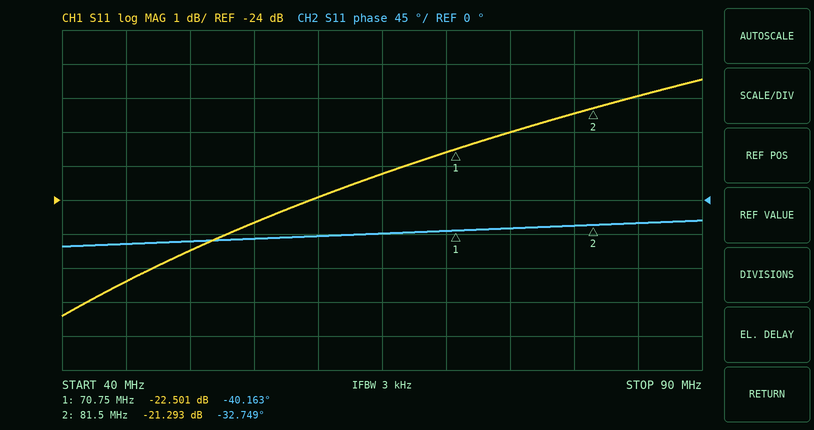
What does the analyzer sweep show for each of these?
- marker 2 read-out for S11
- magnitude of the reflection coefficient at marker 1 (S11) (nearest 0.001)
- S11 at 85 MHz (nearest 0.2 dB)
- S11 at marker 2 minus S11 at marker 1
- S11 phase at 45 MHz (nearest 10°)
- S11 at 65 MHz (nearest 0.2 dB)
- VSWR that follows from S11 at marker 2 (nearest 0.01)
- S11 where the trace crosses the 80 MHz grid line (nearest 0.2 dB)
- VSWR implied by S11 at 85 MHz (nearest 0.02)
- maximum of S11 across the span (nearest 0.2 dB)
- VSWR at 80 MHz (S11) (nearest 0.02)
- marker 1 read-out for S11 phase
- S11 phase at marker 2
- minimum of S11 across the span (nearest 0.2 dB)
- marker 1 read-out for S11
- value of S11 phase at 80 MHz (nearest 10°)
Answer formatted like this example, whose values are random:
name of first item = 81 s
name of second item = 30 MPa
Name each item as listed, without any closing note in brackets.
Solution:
marker 2 read-out for S11 = -21.293 dB
magnitude of the reflection coefficient at marker 1 (S11) = 0.075
S11 at 85 MHz = -21.0 dB
S11 at marker 2 minus S11 at marker 1 = 1.208 dB
S11 phase at 45 MHz = -60°
S11 at 65 MHz = -23.2 dB
VSWR that follows from S11 at marker 2 = 1.19
S11 where the trace crosses the 80 MHz grid line = -21.4 dB
VSWR implied by S11 at 85 MHz = 1.20
maximum of S11 across the span = -20.4 dB
VSWR at 80 MHz (S11) = 1.18
marker 1 read-out for S11 phase = -40.163°
S11 phase at marker 2 = -32.749°
minimum of S11 across the span = -27.4 dB
marker 1 read-out for S11 = -22.501 dB
value of S11 phase at 80 MHz = -30°
